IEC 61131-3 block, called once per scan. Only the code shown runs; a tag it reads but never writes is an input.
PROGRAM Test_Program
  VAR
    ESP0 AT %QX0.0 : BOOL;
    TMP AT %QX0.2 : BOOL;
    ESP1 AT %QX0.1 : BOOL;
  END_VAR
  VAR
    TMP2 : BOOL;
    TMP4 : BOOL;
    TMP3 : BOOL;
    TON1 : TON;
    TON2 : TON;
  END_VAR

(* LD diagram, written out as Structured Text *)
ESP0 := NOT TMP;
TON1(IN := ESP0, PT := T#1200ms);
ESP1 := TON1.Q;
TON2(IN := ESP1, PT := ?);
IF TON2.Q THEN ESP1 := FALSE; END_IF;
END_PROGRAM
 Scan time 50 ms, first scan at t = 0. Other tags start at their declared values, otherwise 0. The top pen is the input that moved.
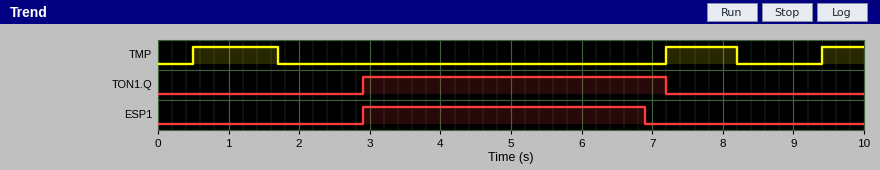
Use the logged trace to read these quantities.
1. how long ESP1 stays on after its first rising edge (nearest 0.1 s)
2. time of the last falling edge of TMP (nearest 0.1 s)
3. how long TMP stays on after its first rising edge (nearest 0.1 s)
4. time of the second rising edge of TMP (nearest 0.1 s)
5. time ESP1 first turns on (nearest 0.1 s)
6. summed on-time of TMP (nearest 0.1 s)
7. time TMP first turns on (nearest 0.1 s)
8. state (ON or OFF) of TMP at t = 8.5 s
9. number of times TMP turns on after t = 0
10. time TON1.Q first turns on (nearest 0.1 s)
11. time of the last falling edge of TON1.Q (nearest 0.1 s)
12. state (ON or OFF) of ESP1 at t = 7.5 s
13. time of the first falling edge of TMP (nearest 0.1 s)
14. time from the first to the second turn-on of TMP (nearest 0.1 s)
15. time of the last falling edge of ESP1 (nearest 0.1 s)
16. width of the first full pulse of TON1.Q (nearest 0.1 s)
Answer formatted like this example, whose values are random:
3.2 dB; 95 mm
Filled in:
4.0 s; 8.2 s; 1.2 s; 7.2 s; 2.9 s; 2.8 s; 0.5 s; OFF; 3; 2.9 s; 7.2 s; OFF; 1.7 s; 6.7 s; 6.9 s; 4.3 s
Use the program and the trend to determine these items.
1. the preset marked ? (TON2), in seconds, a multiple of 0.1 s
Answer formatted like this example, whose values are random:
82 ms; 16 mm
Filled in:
4.0 s
